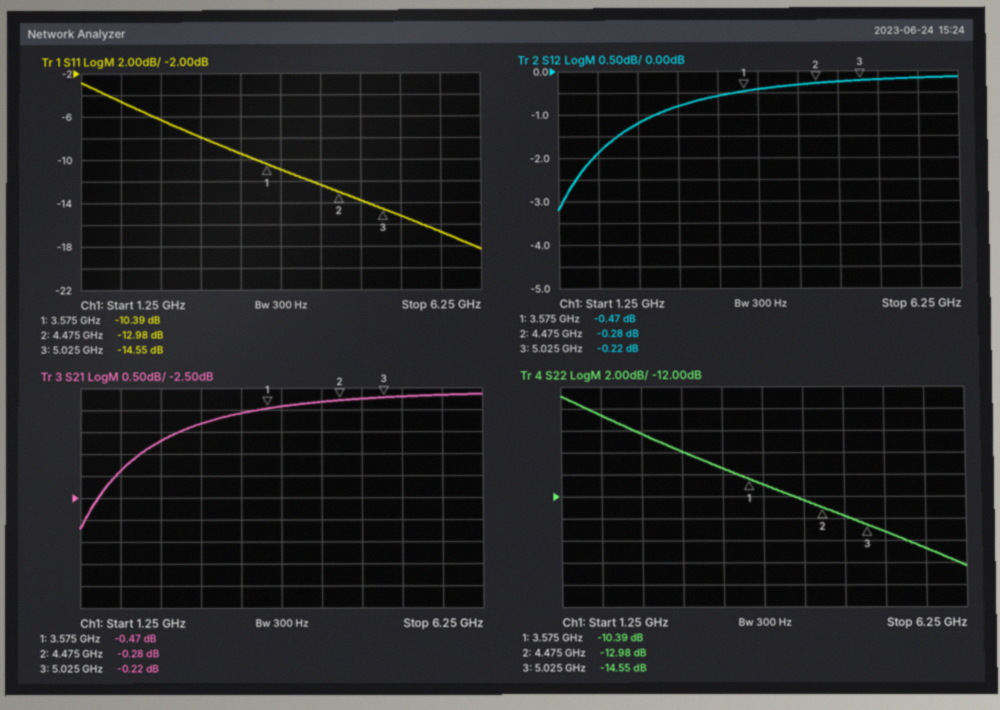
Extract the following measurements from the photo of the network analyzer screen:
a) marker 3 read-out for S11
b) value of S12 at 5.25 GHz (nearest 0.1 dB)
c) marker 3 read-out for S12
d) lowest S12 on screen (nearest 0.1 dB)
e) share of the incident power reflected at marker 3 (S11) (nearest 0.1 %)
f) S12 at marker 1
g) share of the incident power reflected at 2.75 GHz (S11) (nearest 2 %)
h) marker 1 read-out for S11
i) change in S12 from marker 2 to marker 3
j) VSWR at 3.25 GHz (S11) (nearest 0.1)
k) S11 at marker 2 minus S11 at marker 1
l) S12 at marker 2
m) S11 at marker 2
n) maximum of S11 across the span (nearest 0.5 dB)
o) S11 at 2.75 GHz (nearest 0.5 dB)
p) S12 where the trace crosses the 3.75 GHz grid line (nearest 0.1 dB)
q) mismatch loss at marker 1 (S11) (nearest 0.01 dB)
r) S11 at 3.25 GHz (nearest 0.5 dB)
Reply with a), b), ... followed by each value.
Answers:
a) -14.55 dB
b) -0.2 dB
c) -0.22 dB
d) -3.2 dB
e) 3.5 %
f) -0.47 dB
g) 16 %
h) -10.39 dB
i) 0.06 dB
j) 2.0
k) -2.59 dB
l) -0.28 dB
m) -12.98 dB
n) -3.0 dB
o) -8.0 dB
p) -0.4 dB
q) 0.42 dB
r) -9.5 dB
